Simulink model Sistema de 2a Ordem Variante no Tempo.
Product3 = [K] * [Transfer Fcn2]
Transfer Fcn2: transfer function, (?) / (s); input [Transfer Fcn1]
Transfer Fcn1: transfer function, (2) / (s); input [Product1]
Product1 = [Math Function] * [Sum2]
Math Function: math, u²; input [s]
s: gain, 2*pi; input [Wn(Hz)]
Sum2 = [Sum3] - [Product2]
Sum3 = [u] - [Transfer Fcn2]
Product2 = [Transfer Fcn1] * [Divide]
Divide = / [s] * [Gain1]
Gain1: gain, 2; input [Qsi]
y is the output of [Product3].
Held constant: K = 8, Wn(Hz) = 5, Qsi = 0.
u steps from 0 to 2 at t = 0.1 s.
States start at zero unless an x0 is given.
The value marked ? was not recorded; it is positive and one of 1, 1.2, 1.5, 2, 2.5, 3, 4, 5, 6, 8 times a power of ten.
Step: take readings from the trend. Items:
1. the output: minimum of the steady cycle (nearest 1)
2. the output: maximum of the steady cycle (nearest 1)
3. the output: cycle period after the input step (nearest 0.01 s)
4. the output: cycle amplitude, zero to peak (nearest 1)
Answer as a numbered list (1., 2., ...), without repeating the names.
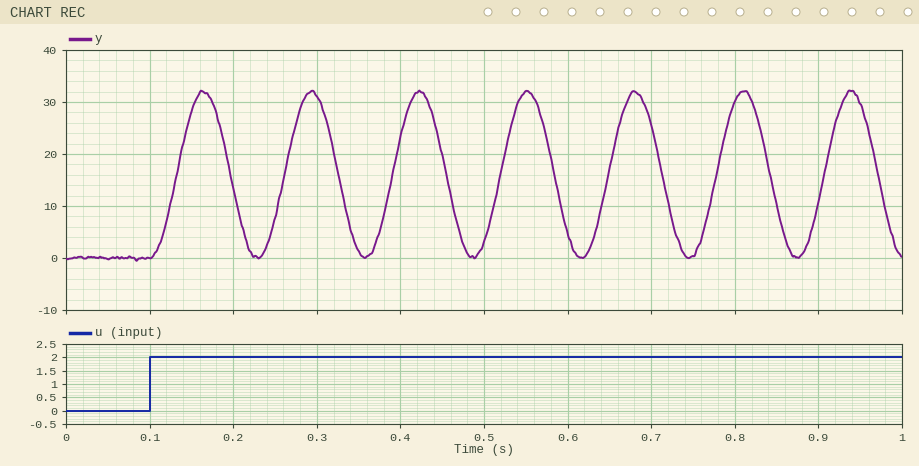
1. 0
2. 32
3. 0.13 s
4. 16
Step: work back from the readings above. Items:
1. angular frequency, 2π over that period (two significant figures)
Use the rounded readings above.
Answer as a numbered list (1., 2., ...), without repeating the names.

1. 48 rad/s
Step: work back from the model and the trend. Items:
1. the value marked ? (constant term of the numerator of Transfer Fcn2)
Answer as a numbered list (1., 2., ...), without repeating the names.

1. 1.2
